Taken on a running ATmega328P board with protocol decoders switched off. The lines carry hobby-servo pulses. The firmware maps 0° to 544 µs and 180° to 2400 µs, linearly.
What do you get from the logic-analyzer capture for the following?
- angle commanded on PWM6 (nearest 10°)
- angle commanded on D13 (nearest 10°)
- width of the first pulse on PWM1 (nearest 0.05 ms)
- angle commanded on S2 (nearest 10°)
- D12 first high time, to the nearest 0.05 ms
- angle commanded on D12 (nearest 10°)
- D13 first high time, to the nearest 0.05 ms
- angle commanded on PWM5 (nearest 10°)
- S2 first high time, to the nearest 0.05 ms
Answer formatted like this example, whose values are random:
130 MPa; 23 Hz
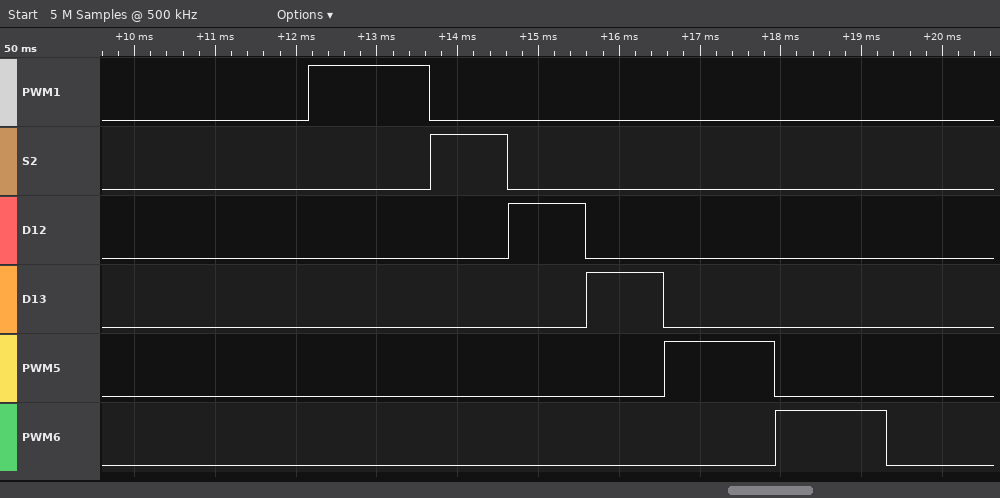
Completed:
80°; 40°; 1.50 ms; 40°; 0.95 ms; 40°; 0.95 ms; 80°; 0.95 ms
